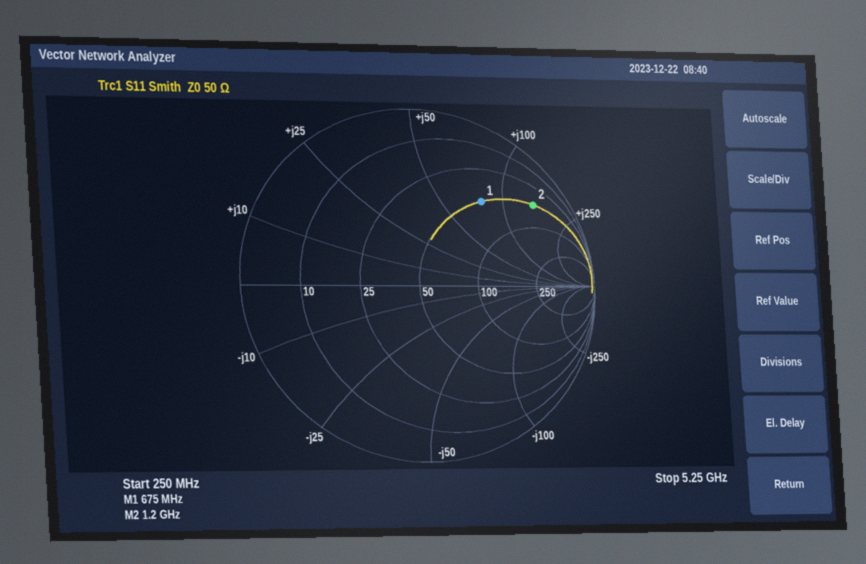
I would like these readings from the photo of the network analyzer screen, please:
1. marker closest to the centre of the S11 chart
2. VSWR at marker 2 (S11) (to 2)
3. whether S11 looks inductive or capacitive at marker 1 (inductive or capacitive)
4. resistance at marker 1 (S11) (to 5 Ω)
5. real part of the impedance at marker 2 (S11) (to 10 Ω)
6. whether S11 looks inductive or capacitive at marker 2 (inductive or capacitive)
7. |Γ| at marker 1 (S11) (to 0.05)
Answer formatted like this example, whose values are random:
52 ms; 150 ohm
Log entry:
marker 1; 10; inductive; 50 Ω; 50 Ω; inductive; 0.60
